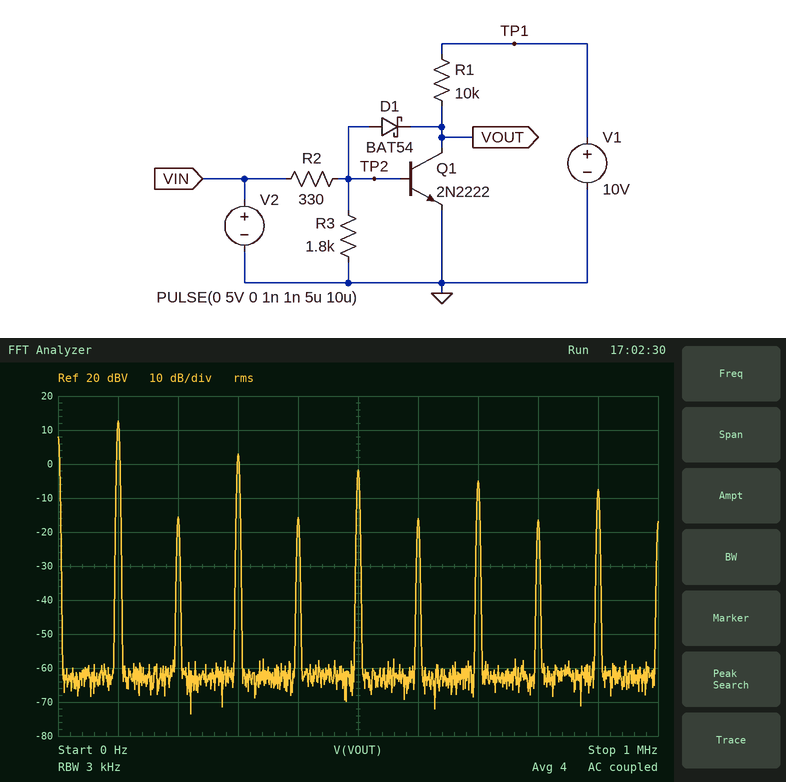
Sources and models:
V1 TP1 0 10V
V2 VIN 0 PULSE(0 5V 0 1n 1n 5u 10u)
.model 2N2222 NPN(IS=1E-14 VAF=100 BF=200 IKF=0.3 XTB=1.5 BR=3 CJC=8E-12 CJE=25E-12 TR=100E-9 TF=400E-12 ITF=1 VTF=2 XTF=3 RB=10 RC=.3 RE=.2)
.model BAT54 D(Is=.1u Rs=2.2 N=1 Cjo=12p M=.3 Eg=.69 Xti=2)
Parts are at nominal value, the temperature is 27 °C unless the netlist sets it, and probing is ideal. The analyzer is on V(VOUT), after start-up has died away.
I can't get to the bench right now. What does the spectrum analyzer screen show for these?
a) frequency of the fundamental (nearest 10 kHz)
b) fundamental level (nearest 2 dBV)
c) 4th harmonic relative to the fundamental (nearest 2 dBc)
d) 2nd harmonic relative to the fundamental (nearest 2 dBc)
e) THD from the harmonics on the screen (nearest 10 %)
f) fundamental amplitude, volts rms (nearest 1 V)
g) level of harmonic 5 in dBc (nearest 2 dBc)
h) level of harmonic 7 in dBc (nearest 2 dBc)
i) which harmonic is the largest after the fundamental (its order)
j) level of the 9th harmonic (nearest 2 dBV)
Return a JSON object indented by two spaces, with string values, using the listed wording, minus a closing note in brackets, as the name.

{
  "frequency of the fundamental": "100 kHz",
  "fundamental level": "12 dBV",
  "4th harmonic relative to the fundamental": "-28 dBc",
  "2nd harmonic relative to the fundamental": "-28 dBc",
  "THD from the harmonics on the screen": "40 %",
  "fundamental amplitude, volts rms": "4 V",
  "level of harmonic 5 in dBc": "-14 dBc",
  "level of harmonic 7 in dBc": "-18 dBc",
  "which harmonic is the largest after the fundamental": "3",
  "level of the 9th harmonic": "-8 dBV"
}
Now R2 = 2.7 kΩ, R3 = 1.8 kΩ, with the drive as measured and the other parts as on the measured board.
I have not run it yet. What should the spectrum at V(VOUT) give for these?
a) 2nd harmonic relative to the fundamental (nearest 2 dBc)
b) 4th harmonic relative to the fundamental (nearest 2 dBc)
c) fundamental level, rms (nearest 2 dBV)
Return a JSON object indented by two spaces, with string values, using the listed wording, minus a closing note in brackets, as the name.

{
  "2nd harmonic relative to the fundamental": "-30 dBc",
  "4th harmonic relative to the fundamental": "-30 dBc",
  "fundamental level, rms": "12 dBV"
}
